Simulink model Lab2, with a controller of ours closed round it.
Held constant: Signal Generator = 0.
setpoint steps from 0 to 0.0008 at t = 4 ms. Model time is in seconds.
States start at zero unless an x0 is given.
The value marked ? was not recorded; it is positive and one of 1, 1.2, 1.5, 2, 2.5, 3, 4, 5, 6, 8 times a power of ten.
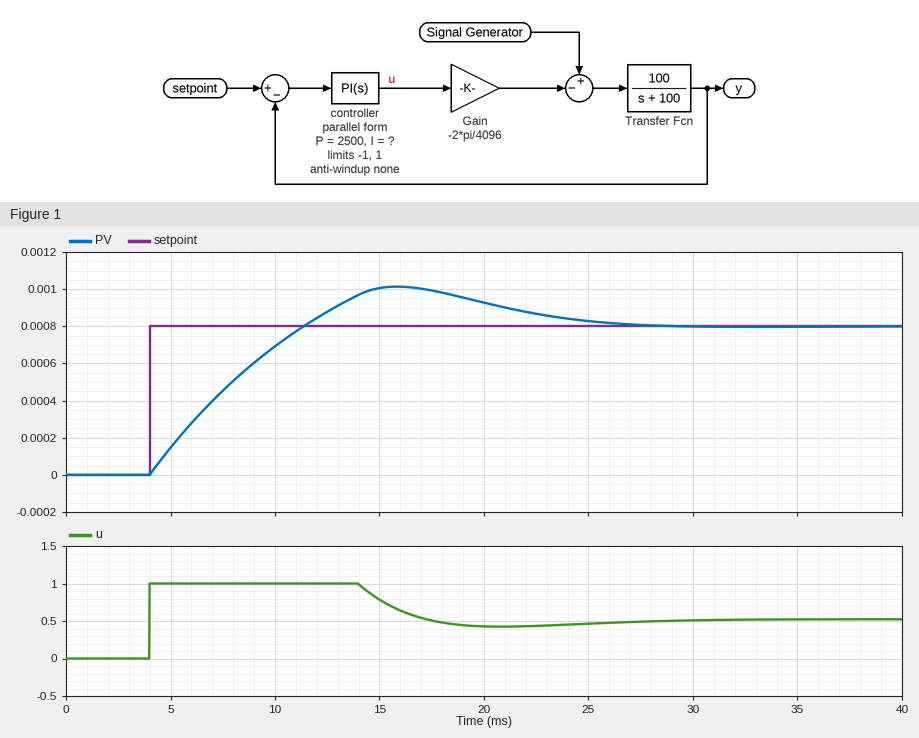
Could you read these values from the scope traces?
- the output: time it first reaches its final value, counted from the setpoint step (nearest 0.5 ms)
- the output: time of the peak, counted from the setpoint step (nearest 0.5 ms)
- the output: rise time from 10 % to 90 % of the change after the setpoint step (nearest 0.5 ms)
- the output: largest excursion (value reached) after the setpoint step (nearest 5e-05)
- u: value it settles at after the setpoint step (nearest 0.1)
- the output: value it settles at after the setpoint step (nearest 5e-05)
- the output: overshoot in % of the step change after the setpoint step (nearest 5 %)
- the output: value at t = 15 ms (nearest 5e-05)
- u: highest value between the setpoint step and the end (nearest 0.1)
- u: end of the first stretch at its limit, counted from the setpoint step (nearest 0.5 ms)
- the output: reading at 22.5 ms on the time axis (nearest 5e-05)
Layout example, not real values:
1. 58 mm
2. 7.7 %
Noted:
1. 7.5 ms
2. 12.0 ms
3. 6.0 ms
4. 0.00100
5. 0.5
6. 0.00080
7. 25 %
8. 0.00100
9. 1.0
10. 10.0 ms
11. 0.00085
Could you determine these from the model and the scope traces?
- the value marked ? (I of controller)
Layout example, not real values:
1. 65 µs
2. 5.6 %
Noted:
1. 600000
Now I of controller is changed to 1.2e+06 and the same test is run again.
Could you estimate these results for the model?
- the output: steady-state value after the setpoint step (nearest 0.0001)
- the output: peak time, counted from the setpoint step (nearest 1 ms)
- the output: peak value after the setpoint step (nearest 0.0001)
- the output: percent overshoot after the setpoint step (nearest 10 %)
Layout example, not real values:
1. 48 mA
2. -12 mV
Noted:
1. 0.0008
2. 14 ms
3. 0.0011
4. 40 %
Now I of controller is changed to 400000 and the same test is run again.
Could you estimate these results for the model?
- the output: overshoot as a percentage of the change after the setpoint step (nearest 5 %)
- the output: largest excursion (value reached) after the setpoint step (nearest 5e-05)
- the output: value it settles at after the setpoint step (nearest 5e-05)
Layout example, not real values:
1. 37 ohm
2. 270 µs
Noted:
1. 15 %
2. 0.00090
3. 0.00080
